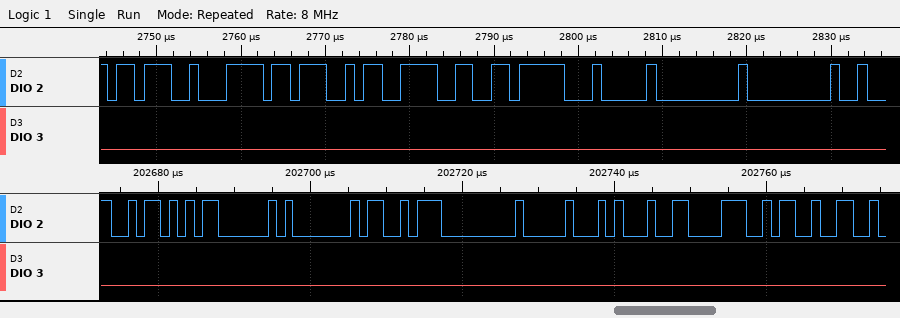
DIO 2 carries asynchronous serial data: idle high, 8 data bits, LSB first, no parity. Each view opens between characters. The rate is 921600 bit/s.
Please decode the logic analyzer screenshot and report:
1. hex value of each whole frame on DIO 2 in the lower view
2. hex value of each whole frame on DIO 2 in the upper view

5A, 03, 01, D3, 00, 10, 91, 38, 93
3B, BC, A7, 9E, F6, 04, 00, 00
